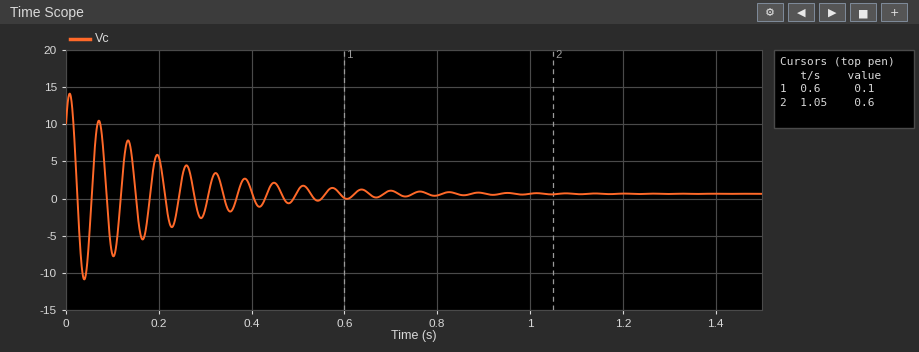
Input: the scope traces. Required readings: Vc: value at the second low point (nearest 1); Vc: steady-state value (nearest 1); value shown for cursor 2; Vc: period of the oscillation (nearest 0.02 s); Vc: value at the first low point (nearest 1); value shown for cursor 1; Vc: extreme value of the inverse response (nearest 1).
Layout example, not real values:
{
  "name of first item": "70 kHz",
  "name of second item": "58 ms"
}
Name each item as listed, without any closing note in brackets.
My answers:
{
  "Vc: value at the second low point": "-8",
  "Vc: steady-state value": "1",
  "value shown for cursor 2": "0.6",
  "Vc: period of the oscillation": "0.06 s",
  "Vc: value at the first low point": "-11",
  "value shown for cursor 1": "0.1",
  "Vc: extreme value of the inverse response": "14"
}
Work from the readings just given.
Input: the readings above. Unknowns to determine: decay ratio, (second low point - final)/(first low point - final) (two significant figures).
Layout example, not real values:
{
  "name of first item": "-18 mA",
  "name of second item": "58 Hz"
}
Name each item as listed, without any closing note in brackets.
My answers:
{
  "decay ratio, (second low point - final)/(first low point - final)": "0.75"
}
